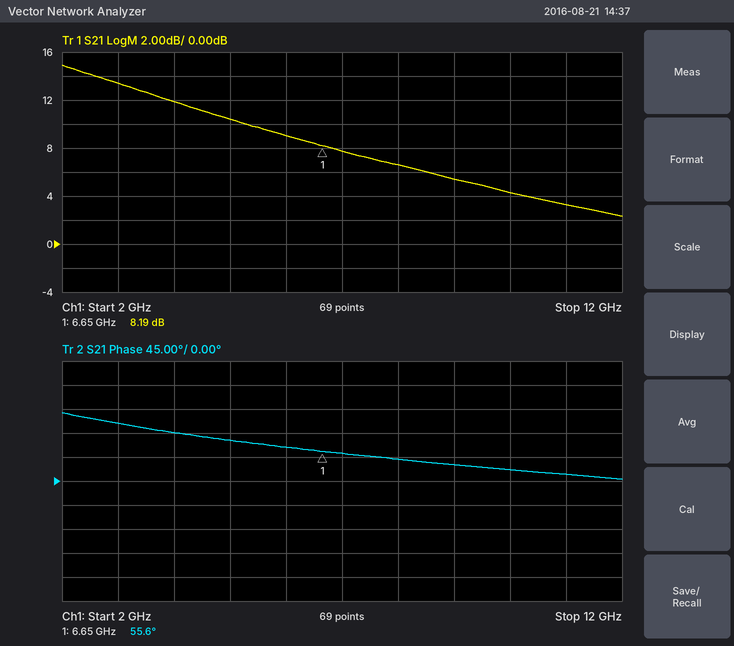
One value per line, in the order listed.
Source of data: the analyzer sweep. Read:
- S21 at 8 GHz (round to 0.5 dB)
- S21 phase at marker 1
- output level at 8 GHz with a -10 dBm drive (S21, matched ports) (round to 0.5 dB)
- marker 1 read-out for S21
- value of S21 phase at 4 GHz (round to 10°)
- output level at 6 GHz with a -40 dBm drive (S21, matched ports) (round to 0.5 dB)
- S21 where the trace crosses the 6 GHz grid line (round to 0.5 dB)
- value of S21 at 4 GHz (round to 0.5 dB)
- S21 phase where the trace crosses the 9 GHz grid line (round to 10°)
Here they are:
6.5 dB
55.6°
-3.5 dBm
8.19 dB
90°
-31.0 dBm
9.0 dB
12.0 dB
30°
